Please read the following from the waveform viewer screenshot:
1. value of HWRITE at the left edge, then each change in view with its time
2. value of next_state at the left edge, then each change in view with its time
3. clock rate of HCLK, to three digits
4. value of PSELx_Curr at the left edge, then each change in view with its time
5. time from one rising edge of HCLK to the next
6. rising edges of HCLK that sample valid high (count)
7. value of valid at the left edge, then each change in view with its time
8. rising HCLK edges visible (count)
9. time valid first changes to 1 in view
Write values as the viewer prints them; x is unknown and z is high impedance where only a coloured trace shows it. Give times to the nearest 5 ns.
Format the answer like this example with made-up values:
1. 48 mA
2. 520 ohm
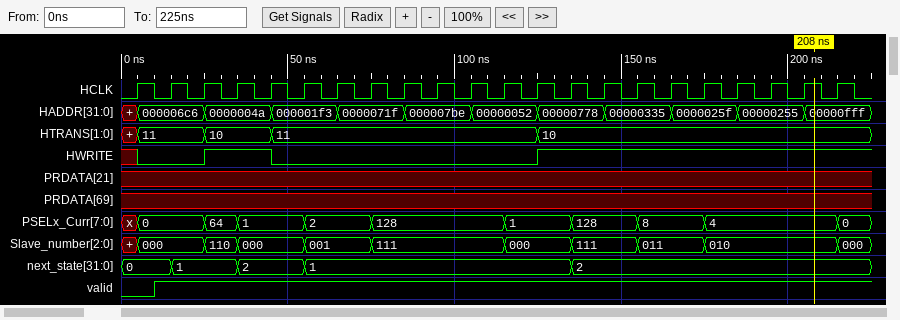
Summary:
1. x, 0 at 5 ns, 1 at 25 ns, 0 at 45 ns, 1 at 125 ns
2. 0, 1 at 15 ns, 2 at 35 ns, 1 at 55 ns, 2 at 135 ns
3. 100 MHz
4. x, 0 at 5 ns, 64 at 25 ns, 1 at 35 ns, 2 at 55 ns, 128 at 75 ns, 1 at 115 ns, 128 at 135 ns, 8 at 155 ns, 4 at 175 ns, 0 at 215 ns
5. 10 ns
6. 21
7. 0, 1 at 10 ns
8. 22
9. 10 ns
